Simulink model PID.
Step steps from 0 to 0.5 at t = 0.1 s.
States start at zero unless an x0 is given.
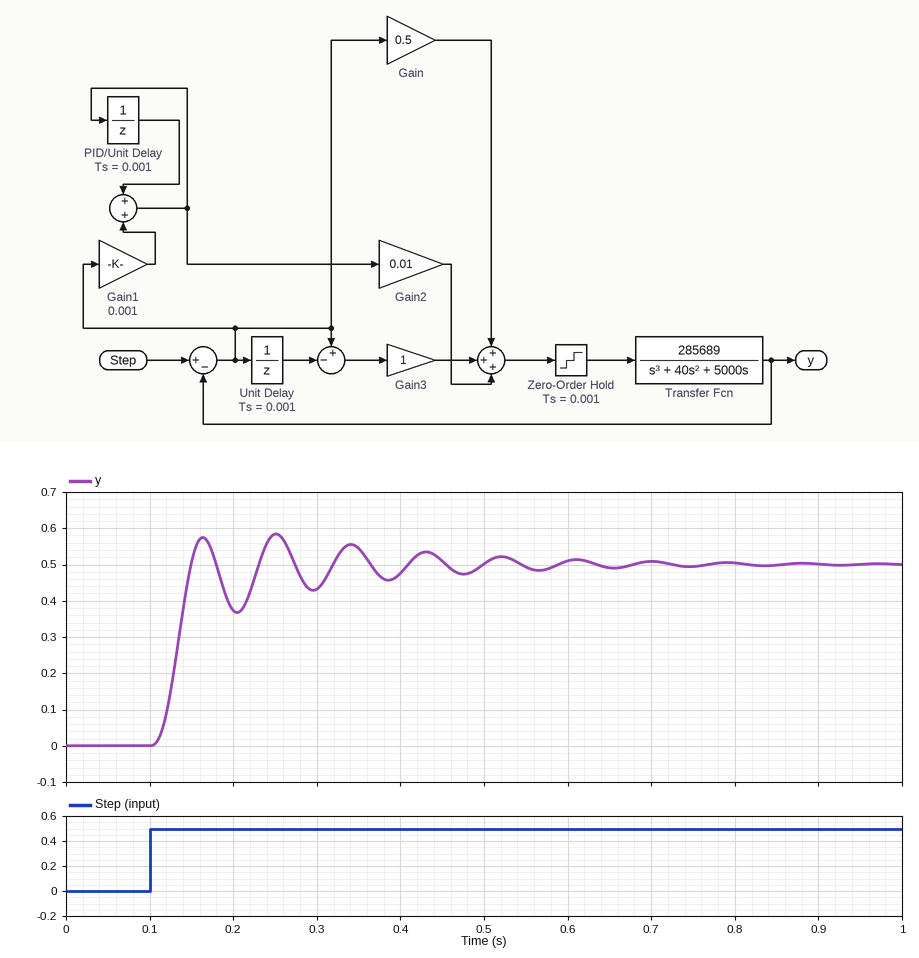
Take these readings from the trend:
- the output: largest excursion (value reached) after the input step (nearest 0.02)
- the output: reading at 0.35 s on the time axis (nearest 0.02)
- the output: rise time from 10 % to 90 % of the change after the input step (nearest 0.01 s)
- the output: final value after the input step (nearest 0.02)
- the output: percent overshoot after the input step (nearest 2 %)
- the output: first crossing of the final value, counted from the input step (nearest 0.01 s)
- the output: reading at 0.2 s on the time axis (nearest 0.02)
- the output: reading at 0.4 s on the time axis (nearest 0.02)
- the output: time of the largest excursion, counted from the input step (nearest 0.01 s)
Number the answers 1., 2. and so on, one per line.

1. 0.58
2. 0.54
3. 0.03 s
4. 0.50
5. 16 %
6. 0.05 s
7. 0.38
8. 0.48
9. 0.15 s
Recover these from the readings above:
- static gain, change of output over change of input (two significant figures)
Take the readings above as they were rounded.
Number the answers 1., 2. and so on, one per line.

1. 1.0
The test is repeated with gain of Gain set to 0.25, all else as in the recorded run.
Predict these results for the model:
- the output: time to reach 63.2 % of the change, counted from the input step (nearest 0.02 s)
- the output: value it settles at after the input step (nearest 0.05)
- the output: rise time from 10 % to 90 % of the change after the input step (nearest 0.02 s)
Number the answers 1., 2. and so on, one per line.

1. 0.06 s
2. 0.50
3. 0.12 s
